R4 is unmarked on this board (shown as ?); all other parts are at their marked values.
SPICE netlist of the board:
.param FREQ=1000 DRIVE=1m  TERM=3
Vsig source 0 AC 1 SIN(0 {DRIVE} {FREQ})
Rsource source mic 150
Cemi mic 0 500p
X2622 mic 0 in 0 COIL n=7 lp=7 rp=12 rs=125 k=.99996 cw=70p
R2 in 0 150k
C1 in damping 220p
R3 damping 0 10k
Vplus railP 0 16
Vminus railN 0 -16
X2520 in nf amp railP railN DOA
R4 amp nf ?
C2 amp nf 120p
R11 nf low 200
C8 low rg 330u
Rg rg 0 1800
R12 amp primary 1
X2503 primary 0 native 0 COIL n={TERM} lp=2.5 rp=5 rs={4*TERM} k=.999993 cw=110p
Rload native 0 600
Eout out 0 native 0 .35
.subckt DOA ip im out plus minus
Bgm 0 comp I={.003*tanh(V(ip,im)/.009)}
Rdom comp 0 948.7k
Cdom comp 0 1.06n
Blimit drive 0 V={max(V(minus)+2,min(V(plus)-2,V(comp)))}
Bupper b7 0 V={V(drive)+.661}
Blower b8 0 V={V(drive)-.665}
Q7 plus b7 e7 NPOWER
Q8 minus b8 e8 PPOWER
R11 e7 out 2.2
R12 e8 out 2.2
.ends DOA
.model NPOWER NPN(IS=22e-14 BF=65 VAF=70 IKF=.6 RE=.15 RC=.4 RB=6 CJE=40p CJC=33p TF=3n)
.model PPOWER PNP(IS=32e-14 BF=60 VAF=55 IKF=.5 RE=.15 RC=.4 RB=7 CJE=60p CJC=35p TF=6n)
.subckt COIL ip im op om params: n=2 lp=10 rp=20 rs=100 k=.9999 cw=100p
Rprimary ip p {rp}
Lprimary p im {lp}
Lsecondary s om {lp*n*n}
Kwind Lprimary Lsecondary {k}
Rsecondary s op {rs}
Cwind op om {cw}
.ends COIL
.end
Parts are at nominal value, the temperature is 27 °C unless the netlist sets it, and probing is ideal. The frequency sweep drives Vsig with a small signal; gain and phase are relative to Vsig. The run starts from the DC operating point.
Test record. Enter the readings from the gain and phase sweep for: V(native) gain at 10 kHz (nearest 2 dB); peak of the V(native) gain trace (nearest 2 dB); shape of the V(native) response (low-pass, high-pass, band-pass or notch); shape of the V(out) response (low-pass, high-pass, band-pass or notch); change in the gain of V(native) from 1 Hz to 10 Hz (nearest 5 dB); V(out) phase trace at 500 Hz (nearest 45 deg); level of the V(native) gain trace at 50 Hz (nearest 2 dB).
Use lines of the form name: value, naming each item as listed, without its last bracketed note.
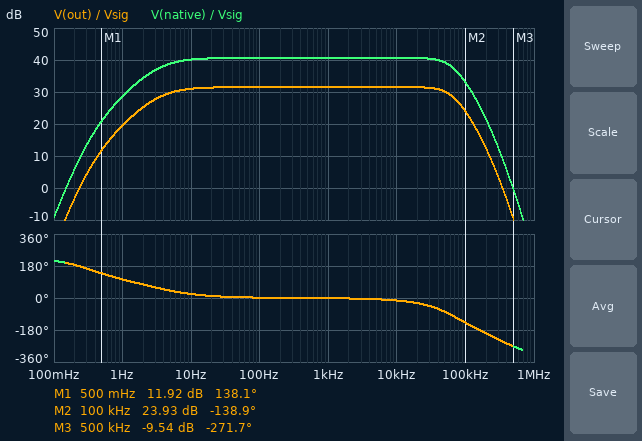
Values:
V(native) gain at 10 kHz: 40 dB
peak of the V(native) gain trace: 40 dB
shape of the V(native) response: band-pass
shape of the V(out) response: band-pass
change in the gain of V(native) from 1 Hz to 10 Hz: 10 dB
V(out) phase trace at 500 Hz: 0 deg
level of the V(native) gain trace at 50 Hz: 40 dB
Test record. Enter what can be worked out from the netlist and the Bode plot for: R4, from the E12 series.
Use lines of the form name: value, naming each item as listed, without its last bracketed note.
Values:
R4, from the E12 series: 10 kΩ
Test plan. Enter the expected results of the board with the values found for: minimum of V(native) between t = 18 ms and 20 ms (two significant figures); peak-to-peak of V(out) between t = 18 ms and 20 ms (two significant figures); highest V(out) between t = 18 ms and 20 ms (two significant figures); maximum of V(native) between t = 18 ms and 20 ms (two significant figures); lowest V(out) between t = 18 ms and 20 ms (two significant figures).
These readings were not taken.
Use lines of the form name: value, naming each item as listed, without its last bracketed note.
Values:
minimum of V(native) between t = 18 ms and 20 ms: -110 mV
peak-to-peak of V(out) between t = 18 ms and 20 ms: 75 mV
highest V(out) between t = 18 ms and 20 ms: 38 mV
maximum of V(native) between t = 18 ms and 20 ms: 110 mV
lowest V(out) between t = 18 ms and 20 ms: -38 mV
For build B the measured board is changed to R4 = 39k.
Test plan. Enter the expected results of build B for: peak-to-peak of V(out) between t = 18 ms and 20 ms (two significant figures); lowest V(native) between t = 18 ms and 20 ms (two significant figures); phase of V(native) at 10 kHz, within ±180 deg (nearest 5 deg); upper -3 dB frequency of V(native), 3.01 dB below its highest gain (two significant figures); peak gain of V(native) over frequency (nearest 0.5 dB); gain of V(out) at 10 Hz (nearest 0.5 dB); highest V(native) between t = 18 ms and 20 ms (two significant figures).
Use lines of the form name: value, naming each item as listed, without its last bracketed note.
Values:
peak-to-peak of V(out) between t = 18 ms and 20 ms: 260 mV
lowest V(native) between t = 18 ms and 20 ms: -370 mV
phase of V(native) at 10 kHz, within ±180 deg: -25 deg
upper -3 dB frequency of V(native), 3.01 dB below its highest gain: 33 kHz
peak gain of V(native) over frequency: 51.5 dB
gain of V(out) at 10 Hz: 41.5 dB
highest V(native) between t = 18 ms and 20 ms: 370 mV
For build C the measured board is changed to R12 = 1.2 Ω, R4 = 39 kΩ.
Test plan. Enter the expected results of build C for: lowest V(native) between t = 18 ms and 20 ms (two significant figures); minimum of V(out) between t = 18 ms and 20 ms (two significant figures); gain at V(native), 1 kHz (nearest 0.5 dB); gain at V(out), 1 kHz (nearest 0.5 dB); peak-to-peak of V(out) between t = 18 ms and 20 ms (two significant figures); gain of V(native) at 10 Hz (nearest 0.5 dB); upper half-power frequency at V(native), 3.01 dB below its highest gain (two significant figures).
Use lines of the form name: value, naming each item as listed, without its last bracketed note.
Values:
lowest V(native) between t = 18 ms and 20 ms: -370 mV
minimum of V(out) between t = 18 ms and 20 ms: -130 mV
gain at V(native), 1 kHz: 51.5 dB
gain at V(out), 1 kHz: 42.0 dB
peak-to-peak of V(out) between t = 18 ms and 20 ms: 260 mV
gain of V(native) at 10 Hz: 51.0 dB
upper half-power frequency at V(native), 3.01 dB below its highest gain: 33 kHz
